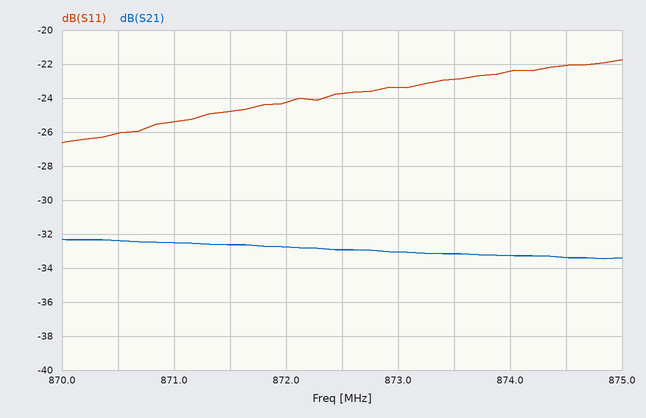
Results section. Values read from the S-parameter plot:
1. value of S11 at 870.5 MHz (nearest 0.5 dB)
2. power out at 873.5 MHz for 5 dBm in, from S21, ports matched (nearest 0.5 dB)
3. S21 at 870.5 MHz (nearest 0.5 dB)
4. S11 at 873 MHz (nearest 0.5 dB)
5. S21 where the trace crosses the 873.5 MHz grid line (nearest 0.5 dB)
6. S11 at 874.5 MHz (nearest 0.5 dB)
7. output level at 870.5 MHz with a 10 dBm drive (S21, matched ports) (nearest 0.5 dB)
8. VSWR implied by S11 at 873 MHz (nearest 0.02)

-26.0 dB
-28.0 dBm
-32.5 dB
-23.5 dB
-33.0 dB
-22.0 dB
-22.5 dBm
1.14
